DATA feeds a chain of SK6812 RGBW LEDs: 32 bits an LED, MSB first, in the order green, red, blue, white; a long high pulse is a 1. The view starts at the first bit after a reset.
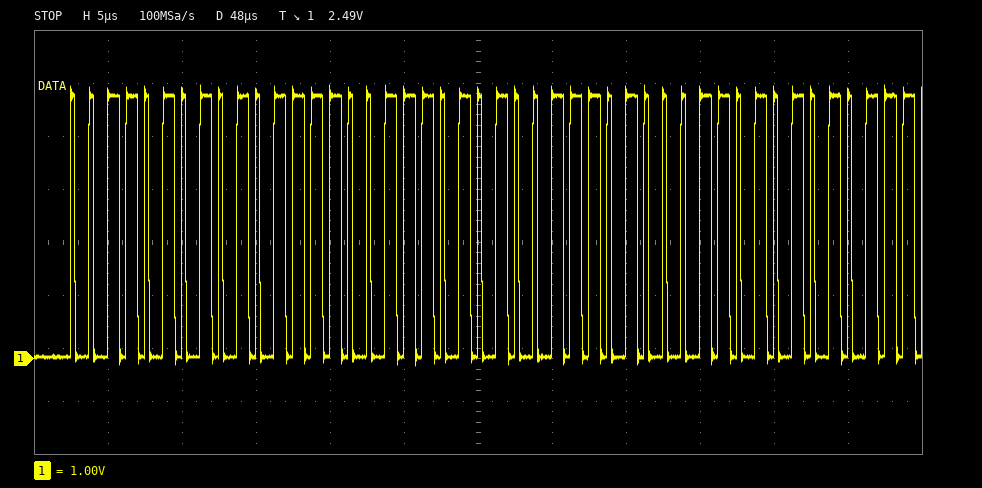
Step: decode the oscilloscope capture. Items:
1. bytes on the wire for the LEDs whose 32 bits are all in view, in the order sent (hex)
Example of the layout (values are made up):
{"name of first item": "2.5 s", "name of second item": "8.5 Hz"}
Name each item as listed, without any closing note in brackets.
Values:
{"bytes on the wire for the LEDs whose 32 bits are all in view, in the order sent": "35 5E 75 3A"}
